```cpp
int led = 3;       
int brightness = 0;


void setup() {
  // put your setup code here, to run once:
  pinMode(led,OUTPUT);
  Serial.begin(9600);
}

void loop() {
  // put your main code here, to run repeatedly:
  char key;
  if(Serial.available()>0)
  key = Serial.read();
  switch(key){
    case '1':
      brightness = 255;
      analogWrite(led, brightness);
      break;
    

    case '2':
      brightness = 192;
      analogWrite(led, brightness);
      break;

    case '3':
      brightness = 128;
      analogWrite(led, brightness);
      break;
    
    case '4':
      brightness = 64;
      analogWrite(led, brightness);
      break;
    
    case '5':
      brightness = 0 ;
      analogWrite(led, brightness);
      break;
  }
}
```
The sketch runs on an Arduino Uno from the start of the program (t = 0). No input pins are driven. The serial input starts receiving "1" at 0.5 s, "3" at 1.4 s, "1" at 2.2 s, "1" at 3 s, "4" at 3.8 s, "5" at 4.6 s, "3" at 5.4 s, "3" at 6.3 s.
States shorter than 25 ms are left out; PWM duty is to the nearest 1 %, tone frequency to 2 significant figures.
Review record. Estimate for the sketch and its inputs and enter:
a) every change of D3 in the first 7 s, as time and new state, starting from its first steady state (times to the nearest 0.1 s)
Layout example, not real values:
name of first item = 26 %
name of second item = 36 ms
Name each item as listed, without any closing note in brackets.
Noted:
every change of D3 in the first 7 s, as time and new state, starting from its first steady state = 0 s low; 0.5 s high; 1.4 s PWM 50 %; 2.2 s high; 3.8 s PWM 25 %; 4.6 s low; 5.4 s PWM 50 %
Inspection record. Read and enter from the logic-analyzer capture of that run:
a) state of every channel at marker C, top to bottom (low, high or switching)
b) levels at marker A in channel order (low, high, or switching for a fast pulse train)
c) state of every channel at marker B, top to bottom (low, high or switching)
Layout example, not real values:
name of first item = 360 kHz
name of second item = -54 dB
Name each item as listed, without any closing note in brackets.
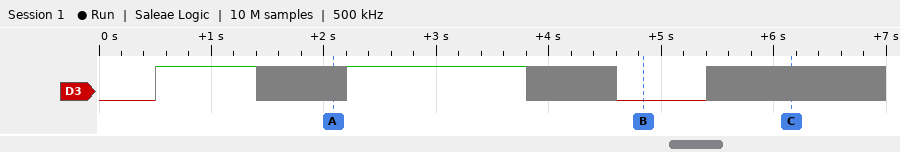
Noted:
state of every channel at marker C, top to bottom = D3 switching
levels at marker A in channel order = D3 switching
state of every channel at marker B, top to bottom = D3 low
